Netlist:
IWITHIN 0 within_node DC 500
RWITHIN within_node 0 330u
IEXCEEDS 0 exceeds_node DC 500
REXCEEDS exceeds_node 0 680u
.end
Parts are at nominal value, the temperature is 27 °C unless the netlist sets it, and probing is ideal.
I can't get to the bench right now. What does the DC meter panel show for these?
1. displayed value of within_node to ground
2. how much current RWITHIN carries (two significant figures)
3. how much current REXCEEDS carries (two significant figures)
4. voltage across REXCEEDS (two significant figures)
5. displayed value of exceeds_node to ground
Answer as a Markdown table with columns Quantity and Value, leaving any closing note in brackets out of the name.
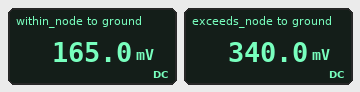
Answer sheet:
| Quantity | Value |
|---|---|
| displayed value of within_node to ground | 165.0 mV |
| how much current RWITHIN carries | 500 A |
| how much current REXCEEDS carries | 500 A |
| voltage across REXCEEDS | 340 mV |
| displayed value of exceeds_node to ground | 340.0 mV |
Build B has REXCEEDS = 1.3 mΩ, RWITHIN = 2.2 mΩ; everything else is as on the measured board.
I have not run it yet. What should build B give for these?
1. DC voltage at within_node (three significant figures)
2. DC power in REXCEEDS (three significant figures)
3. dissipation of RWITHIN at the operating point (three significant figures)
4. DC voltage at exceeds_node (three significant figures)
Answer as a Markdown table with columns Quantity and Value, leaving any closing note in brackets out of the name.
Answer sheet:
| Quantity | Value |
|---|---|
| DC voltage at within_node | 1.10 V |
| DC power in REXCEEDS | 325 W |
| dissipation of RWITHIN at the operating point | 550 W |
| DC voltage at exceeds_node | 650 mV |
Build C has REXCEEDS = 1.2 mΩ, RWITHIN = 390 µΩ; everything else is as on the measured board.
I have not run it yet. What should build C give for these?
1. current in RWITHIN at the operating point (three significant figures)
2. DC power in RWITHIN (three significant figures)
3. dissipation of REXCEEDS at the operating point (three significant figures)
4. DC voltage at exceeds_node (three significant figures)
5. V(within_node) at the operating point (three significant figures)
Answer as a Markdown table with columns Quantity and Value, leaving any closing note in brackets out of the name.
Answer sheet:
| Quantity | Value |
|---|---|
| current in RWITHIN at the operating point | 500 A |
| DC power in RWITHIN | 97.5 W |
| dissipation of REXCEEDS at the operating point | 300 W |
| DC voltage at exceeds_node | 600 mV |
| V(within_node) at the operating point | 195 mV |
